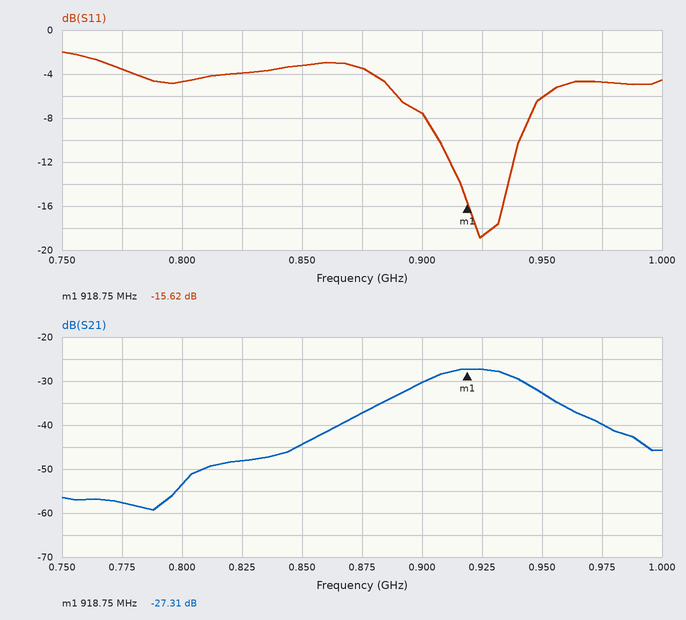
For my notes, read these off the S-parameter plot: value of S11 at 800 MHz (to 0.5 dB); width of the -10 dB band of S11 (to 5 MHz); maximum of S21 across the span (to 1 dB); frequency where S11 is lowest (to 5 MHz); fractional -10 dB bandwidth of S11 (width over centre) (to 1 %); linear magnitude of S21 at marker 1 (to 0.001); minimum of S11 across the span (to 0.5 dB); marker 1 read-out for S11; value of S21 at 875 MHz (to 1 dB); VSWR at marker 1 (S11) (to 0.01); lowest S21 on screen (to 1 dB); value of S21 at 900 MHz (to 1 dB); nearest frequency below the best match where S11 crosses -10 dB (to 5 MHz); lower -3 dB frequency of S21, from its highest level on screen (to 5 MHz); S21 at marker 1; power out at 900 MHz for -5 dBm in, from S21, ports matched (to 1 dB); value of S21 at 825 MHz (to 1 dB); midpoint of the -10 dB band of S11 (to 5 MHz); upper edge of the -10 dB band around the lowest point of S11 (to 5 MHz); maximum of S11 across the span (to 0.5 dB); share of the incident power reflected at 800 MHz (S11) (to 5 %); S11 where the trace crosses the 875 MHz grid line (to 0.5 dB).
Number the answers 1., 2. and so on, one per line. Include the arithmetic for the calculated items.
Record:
1. -4.5 dB
2. 940 MHz − 905 MHz = 35 MHz
3. -27 dB
4. 925 MHz
5. 35 MHz / 922.5 MHz ≈ 4 %
6. 10^(-27.31/20) ≈ 0.043
7. -19.0 dB
8. -15.62 dB
9. -37 dB
10. (1 + 0.1656)/(1 − 0.1656) ≈ 1.40
11. -59 dB
12. -30 dB
13. 905 MHz
14. 900 MHz
15. -27.31 dB
16. -5 dBm + (-30 dB) = -35 dBm
17. -48 dB
18. 925 MHz
19. 940 MHz
20. -2.0 dB
21. 10^(-4.5/10) ≈ 35 %
22. -3.5 dB
